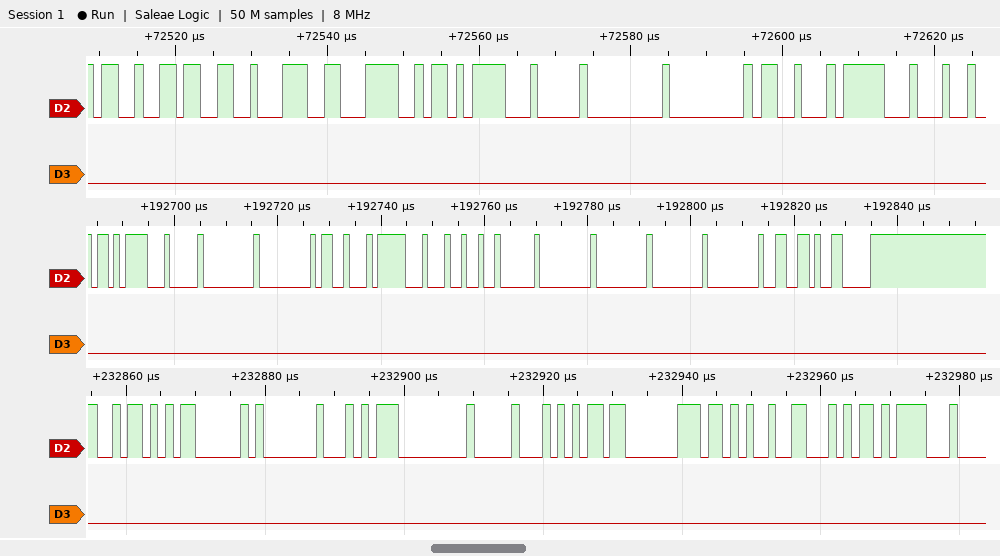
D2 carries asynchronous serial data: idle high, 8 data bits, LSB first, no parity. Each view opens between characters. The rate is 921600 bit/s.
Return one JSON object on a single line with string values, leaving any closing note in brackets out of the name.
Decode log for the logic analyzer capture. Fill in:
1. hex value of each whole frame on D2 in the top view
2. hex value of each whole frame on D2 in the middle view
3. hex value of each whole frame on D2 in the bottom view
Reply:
{"hex value of each whole frame on D2 in the top view": "93, 33, 9C, 3C, EB, 04, 00, 00, 13, 1F", "hex value of each whole frame on D2 in the middle view": "EB, 04, 00, 00, 13, 1F, 24, 02, 00, 00, 00, 00, 66, 06", "hex value of each whole frame on D2 in the bottom view": "5A, 03, 01, D4, 00, 10, B5, C0, 2B, 46, EB"}
